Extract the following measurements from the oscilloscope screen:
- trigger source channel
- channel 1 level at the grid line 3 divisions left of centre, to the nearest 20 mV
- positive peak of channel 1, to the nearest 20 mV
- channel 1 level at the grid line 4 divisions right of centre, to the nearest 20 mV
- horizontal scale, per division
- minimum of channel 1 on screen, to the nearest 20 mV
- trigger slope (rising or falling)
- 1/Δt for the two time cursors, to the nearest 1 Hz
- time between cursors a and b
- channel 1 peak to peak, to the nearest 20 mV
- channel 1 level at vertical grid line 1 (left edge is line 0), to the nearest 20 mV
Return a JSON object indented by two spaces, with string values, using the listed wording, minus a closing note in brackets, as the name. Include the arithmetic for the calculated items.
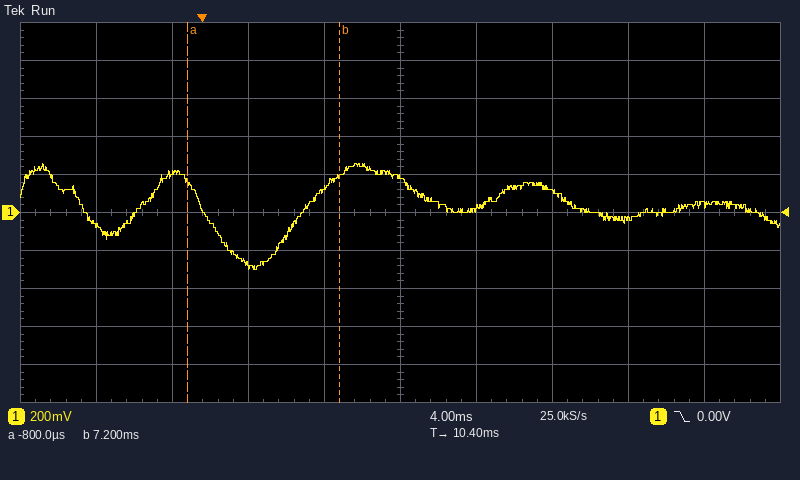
{
  "trigger source channel": "channel 1",
  "channel 1 level at the grid line 3 divisions left of centre, to the nearest 20 mV": "200 mV",
  "positive peak of channel 1, to the nearest 20 mV": "260 mV",
  "channel 1 level at the grid line 4 divisions right of centre, to the nearest 20 mV": "40 mV",
  "horizontal scale, per division": "4 ms",
  "minimum of channel 1 on screen, to the nearest 20 mV": "-300 mV",
  "trigger slope": "falling",
  "1/Δt for the two time cursors, to the nearest 1 Hz": "1 / 8.0 ms ≈ 125 Hz",
  "time between cursors a and b": "7.2 ms − (-800 µs) = 8.0 ms",
  "channel 1 peak to peak, to the nearest 20 mV": "260 mV − (-300 mV) = 560 mV",
  "channel 1 level at vertical grid line 1 (left edge is line 0), to the nearest 20 mV": "-60 mV"
}
